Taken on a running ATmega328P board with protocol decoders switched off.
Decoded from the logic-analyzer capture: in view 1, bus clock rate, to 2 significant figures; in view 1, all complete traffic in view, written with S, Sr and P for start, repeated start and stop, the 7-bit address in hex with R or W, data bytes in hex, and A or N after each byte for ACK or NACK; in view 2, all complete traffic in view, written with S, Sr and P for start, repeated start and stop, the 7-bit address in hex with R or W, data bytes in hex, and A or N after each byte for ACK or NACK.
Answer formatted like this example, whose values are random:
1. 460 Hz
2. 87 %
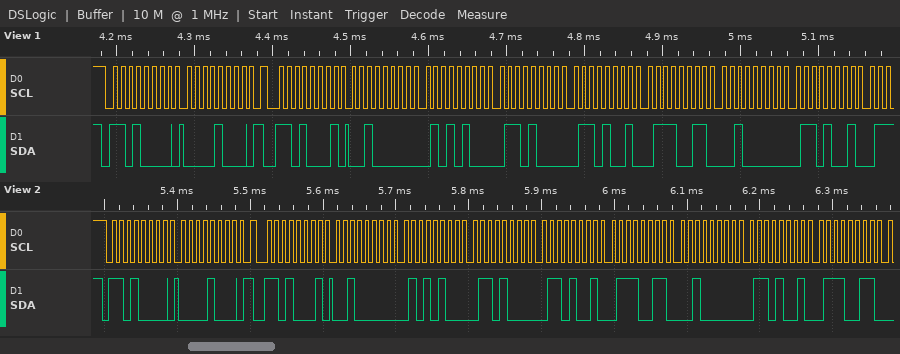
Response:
1. 100 kHz
2. S 68W A 08 A Sr 68R A 20 A 54 A 68 A 69 A 73 A 20 A 69 A
3. S 68W A 08 A Sr 68R A 20 A 54 A 68 A 69 A 73 A 20 A 69 A 73 A
